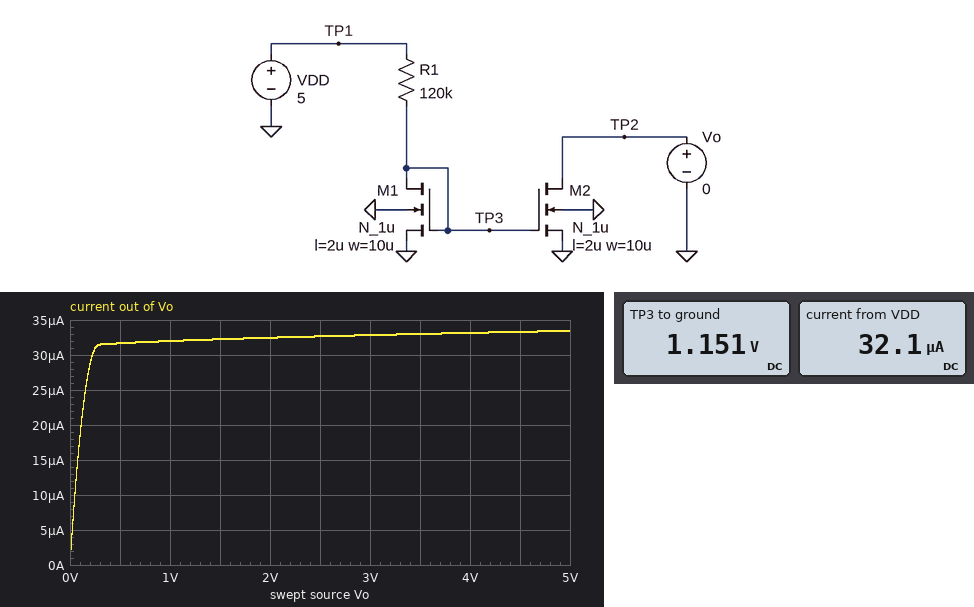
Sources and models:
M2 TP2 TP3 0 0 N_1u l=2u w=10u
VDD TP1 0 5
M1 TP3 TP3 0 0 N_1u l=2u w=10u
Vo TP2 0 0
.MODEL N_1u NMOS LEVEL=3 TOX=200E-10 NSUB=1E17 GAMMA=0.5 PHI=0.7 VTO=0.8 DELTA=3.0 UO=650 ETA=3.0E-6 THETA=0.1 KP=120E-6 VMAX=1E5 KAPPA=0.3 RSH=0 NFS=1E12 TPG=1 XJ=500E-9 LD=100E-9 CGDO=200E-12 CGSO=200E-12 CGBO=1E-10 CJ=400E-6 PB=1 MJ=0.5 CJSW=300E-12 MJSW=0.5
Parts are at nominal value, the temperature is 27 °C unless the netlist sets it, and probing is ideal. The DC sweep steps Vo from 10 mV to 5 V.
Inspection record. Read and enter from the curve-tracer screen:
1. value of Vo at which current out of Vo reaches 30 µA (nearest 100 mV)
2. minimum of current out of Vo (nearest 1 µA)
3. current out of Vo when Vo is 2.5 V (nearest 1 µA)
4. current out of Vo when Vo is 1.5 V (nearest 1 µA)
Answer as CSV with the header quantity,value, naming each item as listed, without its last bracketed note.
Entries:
quantity,value
value of Vo at which current out of Vo reaches 30 µA,200 mV
minimum of current out of Vo,2 µA
current out of Vo when Vo is 2.5 V,33 µA
current out of Vo when Vo is 1.5 V,32 µA
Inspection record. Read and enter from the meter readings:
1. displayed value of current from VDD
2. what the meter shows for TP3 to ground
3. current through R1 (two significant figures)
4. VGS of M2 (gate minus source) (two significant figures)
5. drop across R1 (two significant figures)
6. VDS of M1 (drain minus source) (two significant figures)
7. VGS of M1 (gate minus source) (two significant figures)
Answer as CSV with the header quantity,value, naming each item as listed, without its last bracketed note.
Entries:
quantity,value
displayed value of current from VDD,32.1 µA
what the meter shows for TP3 to ground,1.151 V
current through R1,32 µA
VGS of M2 (gate minus source),1.2 V
drop across R1,3.8 V
VDS of M1 (drain minus source),1.2 V
VGS of M1 (gate minus source),1.2 V
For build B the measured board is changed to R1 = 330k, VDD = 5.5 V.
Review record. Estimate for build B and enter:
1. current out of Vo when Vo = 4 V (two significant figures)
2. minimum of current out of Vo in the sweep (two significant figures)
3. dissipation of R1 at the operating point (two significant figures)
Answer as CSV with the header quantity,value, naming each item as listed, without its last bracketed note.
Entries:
quantity,value
current out of Vo when Vo = 4 V,14 µA
minimum of current out of Vo in the sweep,1.4 µA
dissipation of R1 at the operating point,61 µW
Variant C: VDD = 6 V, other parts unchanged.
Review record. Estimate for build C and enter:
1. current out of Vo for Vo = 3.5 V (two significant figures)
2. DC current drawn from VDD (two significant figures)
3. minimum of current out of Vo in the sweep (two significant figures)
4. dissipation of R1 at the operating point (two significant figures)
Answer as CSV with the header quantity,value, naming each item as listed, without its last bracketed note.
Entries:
quantity,value
current out of Vo for Vo = 3.5 V,41 µA
DC current drawn from VDD,40 µA
minimum of current out of Vo in the sweep,2.5 µA
dissipation of R1 at the operating point,190 µW
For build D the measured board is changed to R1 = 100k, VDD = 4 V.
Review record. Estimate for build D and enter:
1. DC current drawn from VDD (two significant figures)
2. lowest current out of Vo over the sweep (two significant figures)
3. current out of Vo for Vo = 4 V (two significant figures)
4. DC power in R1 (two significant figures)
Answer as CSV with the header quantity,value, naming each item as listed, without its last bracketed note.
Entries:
quantity,value
DC current drawn from VDD,29 µA
lowest current out of Vo over the sweep,2.1 µA
current out of Vo for Vo = 4 V,30 µA
DC power in R1,82 µW
